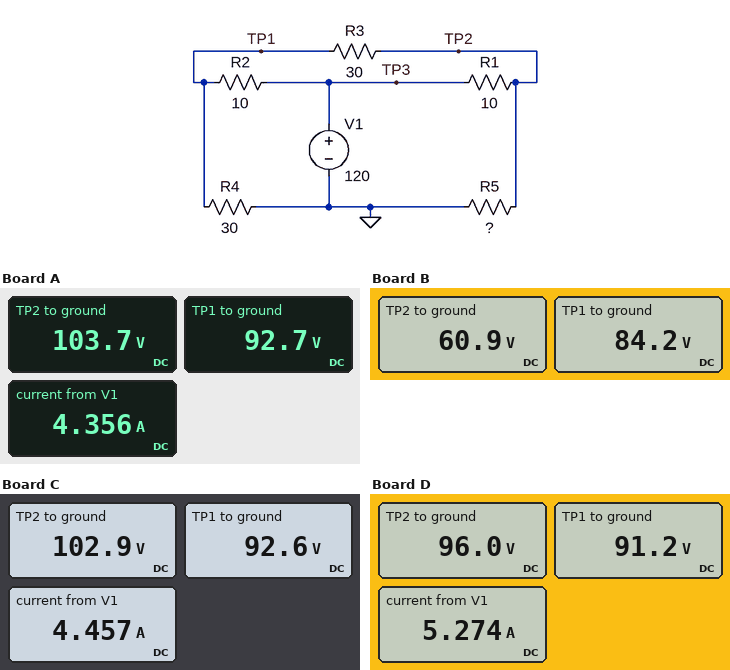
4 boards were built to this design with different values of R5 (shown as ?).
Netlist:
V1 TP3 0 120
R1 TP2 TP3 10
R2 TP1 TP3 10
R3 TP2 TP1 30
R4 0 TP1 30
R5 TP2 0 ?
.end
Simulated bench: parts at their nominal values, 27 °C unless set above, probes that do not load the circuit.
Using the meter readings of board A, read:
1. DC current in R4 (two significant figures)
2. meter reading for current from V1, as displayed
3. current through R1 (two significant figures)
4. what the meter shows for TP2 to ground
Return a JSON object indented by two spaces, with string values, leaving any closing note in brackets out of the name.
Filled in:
{
  "DC current in R4": "3.1 A",
  "meter reading for current from V1, as displayed": "4.356 A",
  "current through R1": "1.6 A",
  "what the meter shows for TP2 to ground": "103.7 V"
}
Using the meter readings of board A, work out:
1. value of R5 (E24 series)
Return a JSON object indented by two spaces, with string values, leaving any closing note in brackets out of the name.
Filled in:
{
  "value of R5": "82 Ω"
}
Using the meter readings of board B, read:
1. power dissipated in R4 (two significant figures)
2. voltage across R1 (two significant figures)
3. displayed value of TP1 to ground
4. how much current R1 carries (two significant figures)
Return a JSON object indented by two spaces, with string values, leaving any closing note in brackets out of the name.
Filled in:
{
  "power dissipated in R4": "240 W",
  "voltage across R1": "59 V",
  "displayed value of TP1 to ground": "84.2 V",
  "how much current R1 carries": "5.9 A"
}
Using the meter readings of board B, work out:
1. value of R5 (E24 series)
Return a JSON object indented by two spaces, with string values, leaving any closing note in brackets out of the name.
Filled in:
{
  "value of R5": "9.1 Ω"
}
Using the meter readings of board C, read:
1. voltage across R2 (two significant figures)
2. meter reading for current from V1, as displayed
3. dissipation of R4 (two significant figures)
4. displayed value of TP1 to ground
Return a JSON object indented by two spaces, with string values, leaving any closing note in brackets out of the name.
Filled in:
{
  "voltage across R2": "27 V",
  "meter reading for current from V1, as displayed": "4.457 A",
  "dissipation of R4": "290 W",
  "displayed value of TP1 to ground": "92.6 V"
}
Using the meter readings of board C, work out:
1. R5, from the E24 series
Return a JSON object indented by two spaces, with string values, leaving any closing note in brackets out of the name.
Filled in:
{
  "R5, from the E24 series": "75 Ω"
}
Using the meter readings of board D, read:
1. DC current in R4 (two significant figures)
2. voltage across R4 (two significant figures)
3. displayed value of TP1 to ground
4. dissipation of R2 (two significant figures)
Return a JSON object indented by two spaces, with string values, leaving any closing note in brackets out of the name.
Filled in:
{
  "DC current in R4": "3.0 A",
  "voltage across R4": "91 V",
  "displayed value of TP1 to ground": "91.2 V",
  "dissipation of R2": "83 W"
}
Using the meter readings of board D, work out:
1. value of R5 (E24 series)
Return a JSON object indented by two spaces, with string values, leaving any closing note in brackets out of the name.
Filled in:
{
  "value of R5": "43 Ω"
}
